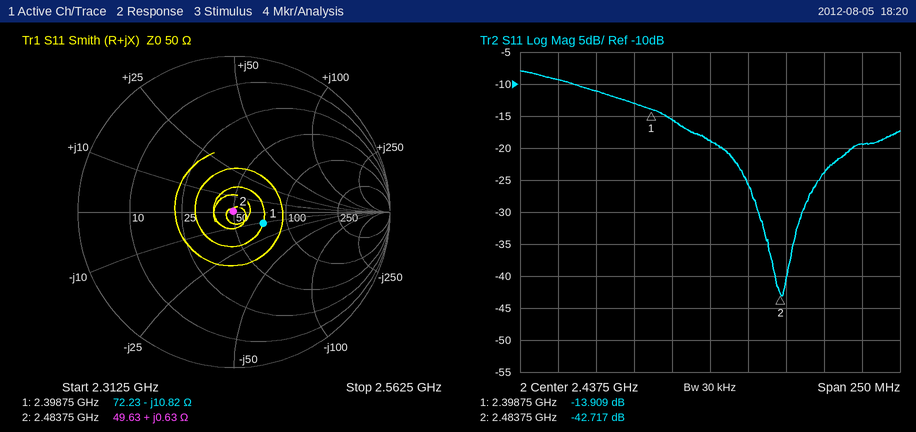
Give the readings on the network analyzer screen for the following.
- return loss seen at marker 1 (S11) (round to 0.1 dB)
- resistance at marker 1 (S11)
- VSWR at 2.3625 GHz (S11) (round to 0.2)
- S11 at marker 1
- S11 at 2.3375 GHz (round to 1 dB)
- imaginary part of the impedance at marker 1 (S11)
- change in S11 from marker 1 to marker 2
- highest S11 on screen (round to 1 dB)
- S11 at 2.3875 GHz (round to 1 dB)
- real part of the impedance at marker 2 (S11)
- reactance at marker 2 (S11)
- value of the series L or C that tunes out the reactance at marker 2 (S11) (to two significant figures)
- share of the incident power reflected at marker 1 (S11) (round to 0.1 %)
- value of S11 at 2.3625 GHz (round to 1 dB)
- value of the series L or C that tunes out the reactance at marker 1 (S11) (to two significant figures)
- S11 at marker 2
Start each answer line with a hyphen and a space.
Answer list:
- 13.9 dB
- 72.23 Ω
- 1.8
- -13.909 dB
- -9 dB
- -10.82 Ω
- -28.808 dB
- -8 dB
- -13 dB
- 49.63 Ω
- +0.63 Ω
- 100 pF
- 4.1 %
- -11 dB
- 720 pH
- -42.717 dB
